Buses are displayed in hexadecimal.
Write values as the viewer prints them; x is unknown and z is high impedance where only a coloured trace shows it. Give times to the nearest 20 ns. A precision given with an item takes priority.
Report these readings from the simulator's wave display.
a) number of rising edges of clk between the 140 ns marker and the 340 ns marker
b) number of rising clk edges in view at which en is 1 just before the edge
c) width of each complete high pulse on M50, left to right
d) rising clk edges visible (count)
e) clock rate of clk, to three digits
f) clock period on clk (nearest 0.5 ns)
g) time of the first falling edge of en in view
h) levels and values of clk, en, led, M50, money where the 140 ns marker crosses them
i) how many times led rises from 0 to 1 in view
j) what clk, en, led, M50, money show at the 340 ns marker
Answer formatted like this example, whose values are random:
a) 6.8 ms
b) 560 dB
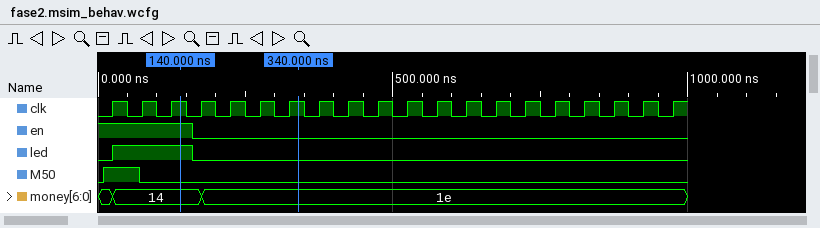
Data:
a) 4
b) 3
c) 60 ns
d) 20
e) 20.0 MHz
f) 50 ns
g) 160 ns
h) clk=1, en=1, led=1, M50=0, money=14
i) 1
j) clk=1, en=0, led=0, M50=0, money=1e
